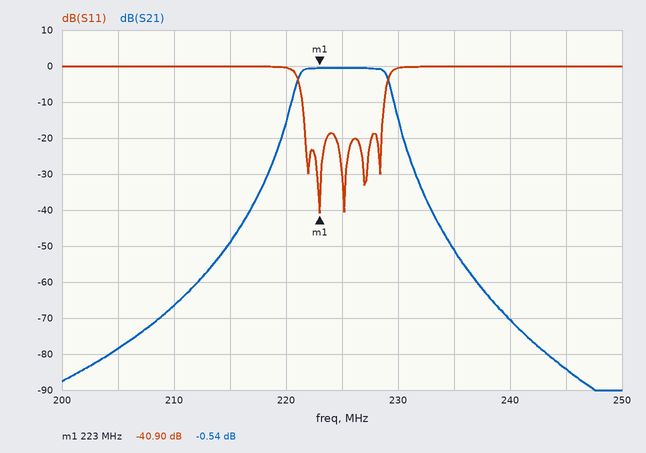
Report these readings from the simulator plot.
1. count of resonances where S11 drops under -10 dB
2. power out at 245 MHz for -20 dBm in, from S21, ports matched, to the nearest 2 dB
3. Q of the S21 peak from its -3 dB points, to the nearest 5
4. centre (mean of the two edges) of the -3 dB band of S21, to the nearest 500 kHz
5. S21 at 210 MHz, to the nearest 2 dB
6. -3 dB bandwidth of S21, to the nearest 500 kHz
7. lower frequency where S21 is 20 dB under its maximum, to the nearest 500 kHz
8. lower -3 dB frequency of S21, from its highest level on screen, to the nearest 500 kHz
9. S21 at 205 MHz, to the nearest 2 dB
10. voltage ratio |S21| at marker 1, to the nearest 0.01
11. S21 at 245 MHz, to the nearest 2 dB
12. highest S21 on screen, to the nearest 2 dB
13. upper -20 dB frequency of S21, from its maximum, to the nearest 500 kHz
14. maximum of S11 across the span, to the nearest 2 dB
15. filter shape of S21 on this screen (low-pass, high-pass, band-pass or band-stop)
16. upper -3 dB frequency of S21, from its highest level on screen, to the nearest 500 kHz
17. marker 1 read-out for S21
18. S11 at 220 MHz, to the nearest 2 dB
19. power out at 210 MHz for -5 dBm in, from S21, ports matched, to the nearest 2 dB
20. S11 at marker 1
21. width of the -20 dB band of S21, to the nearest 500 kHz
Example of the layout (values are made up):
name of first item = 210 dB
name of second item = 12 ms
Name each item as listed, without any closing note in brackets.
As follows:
count of resonances where S11 drops under -10 dB = 5
power out at 245 MHz for -20 dBm in, from S21, ports matched, to the nearest 2 dB = -104 dBm
Q of the S21 peak from its -3 dB points, to the nearest 5 = 30
centre (mean of the two edges) of the -3 dB band of S21, to the nearest 500 kHz = 225.0 MHz
S21 at 210 MHz, to the nearest 2 dB = -66 dB
-3 dB bandwidth of S21, to the nearest 500 kHz = 8.0 MHz
lower frequency where S21 is 20 dB under its maximum, to the nearest 500 kHz = 219.5 MHz
lower -3 dB frequency of S21, from its highest level on screen, to the nearest 500 kHz = 221.0 MHz
S21 at 205 MHz, to the nearest 2 dB = -78 dB
voltage ratio |S21| at marker 1, to the nearest 0.01 = 0.94
S21 at 245 MHz, to the nearest 2 dB = -84 dB
highest S21 on screen, to the nearest 2 dB = 0 dB
upper -20 dB frequency of S21, from its maximum, to the nearest 500 kHz = 230.5 MHz
maximum of S11 across the span, to the nearest 2 dB = 0 dB
filter shape of S21 on this screen = band-pass
upper -3 dB frequency of S21, from its highest level on screen, to the nearest 500 kHz = 229.0 MHz
marker 1 read-out for S21 = -0.54 dB
S11 at 220 MHz, to the nearest 2 dB = 0 dB
power out at 210 MHz for -5 dBm in, from S21, ports matched, to the nearest 2 dB = -72 dBm
S11 at marker 1 = -40.90 dB
width of the -20 dB band of S21, to the nearest 500 kHz = 11.0 MHz
